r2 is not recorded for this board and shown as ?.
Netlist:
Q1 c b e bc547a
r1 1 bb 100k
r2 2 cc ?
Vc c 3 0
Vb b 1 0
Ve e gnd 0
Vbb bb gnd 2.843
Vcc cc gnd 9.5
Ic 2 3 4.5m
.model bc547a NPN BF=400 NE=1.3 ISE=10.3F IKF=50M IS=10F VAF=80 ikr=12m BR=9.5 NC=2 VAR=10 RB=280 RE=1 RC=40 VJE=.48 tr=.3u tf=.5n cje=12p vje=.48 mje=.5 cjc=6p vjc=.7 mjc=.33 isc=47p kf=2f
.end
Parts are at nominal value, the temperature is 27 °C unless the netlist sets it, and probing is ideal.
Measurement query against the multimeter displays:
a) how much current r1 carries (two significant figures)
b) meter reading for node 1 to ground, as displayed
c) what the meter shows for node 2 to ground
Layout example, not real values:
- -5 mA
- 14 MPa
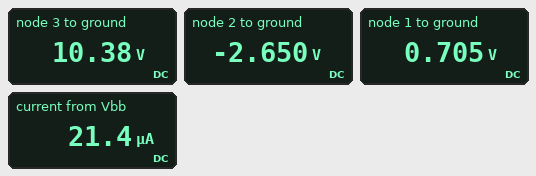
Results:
- 21 µA
- 0.705 V
- -2.650 V
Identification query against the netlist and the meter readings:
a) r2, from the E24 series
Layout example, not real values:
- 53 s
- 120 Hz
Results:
- 2.7 kΩ
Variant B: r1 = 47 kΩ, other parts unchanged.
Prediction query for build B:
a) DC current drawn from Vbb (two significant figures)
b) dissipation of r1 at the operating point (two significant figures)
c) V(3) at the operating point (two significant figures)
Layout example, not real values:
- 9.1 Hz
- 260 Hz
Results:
- 45 µA
- 96 µW
- 280 mV
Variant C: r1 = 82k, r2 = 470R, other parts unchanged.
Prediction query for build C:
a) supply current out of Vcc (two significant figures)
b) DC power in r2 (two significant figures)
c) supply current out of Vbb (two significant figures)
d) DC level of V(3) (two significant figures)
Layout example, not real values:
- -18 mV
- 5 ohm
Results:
- 4.5 mA
- 9.5 mW
- 26 µA
- 360 mV
